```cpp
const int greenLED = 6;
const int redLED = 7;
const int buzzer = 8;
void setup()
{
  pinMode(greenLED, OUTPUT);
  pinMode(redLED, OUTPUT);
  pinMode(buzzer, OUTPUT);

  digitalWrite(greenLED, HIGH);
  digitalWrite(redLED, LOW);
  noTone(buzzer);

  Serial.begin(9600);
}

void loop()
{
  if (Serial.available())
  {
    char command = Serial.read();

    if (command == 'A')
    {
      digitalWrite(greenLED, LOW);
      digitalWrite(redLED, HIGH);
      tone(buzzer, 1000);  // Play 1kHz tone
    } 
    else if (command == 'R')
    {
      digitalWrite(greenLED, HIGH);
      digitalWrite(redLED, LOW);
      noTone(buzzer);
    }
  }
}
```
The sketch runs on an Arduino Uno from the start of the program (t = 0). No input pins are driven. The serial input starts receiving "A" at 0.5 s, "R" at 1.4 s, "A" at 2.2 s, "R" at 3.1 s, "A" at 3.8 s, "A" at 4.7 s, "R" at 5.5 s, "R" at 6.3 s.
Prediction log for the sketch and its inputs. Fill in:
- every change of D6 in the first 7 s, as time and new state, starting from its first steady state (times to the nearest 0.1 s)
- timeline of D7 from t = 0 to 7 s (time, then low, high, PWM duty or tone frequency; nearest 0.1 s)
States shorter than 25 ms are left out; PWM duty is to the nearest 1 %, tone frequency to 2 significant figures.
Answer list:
0 s high; 0.5 s low; 1.4 s high; 2.2 s low; 3.1 s high; 3.8 s low; 5.5 s high
0 s low; 0.5 s high; 1.4 s low; 2.2 s high; 3.1 s low; 3.8 s high; 5.5 s low
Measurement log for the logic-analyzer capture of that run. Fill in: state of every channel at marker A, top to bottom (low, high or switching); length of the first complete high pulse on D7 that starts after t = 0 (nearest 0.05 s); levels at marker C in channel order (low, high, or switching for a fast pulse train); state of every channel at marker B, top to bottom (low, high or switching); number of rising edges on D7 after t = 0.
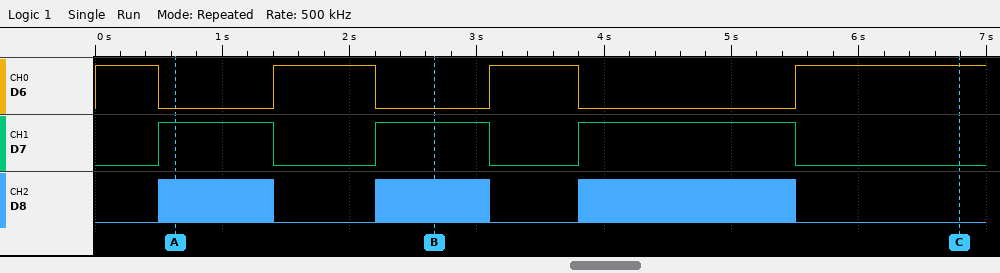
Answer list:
D6 low, D7 high, D8 switching
0.90 s
D6 high, D7 low, D8 low
D6 low, D7 high, D8 switching
3
